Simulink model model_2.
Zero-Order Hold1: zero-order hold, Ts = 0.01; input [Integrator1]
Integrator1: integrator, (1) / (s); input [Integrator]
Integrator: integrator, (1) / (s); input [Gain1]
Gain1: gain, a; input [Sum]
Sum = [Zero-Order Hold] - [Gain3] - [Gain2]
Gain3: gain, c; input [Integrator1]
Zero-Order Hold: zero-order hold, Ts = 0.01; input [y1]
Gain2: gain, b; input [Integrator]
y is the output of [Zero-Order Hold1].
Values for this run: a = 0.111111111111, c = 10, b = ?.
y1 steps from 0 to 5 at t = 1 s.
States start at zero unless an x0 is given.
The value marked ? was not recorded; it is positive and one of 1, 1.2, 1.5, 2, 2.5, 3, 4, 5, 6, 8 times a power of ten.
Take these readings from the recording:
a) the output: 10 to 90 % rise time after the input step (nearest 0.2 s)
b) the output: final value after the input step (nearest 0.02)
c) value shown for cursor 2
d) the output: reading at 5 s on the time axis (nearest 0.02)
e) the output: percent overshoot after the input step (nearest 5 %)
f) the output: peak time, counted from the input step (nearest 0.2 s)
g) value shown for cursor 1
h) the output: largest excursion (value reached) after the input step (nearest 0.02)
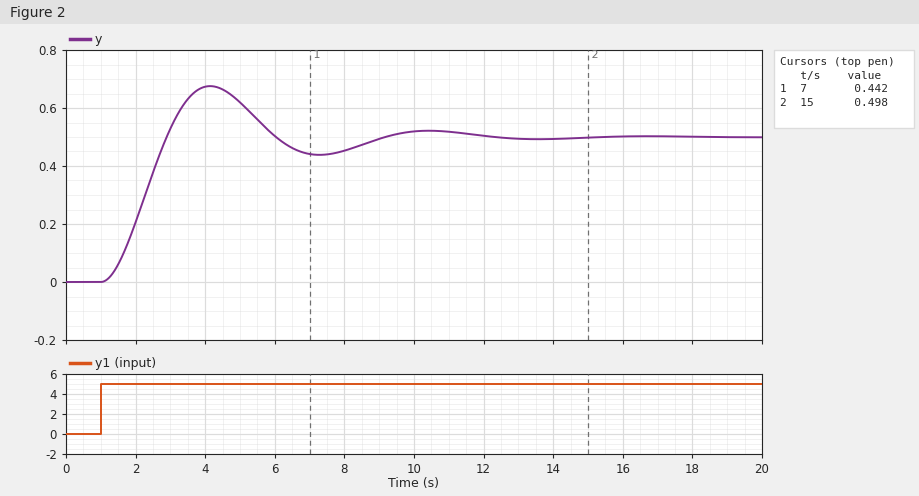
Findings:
1.2 s
0.50
0.498
0.62
35 %
3.2 s
0.442
0.68
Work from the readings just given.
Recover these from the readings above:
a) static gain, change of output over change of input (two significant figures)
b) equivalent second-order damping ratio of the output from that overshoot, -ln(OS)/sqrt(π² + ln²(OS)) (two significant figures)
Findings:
0.10
0.32
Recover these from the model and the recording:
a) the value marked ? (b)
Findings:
6
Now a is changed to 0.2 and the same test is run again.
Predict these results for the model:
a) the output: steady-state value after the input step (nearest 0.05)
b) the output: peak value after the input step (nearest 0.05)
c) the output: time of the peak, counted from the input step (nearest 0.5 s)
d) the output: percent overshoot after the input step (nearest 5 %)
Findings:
0.50
0.60
2.5 s
25 %
